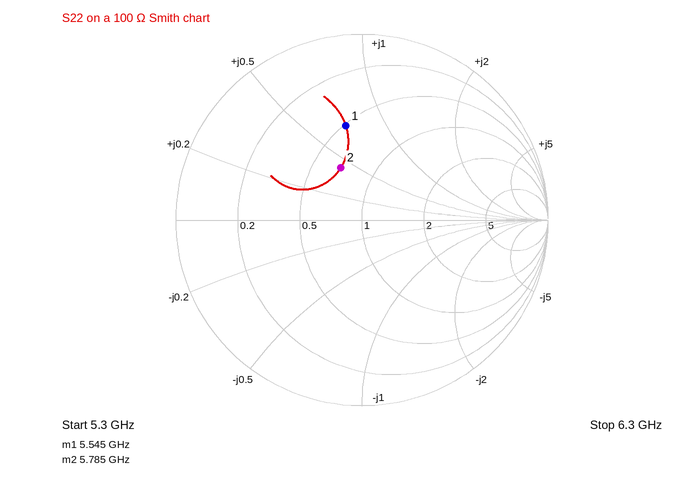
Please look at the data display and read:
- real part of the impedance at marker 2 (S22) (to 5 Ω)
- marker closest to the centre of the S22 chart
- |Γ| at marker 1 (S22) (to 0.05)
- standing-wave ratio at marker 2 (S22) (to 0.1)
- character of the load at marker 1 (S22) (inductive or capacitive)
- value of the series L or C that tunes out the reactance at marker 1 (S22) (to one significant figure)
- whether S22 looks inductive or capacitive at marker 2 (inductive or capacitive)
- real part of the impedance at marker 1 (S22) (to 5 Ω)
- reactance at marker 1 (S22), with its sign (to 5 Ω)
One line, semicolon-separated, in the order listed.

70 Ω; marker 2; 0.50; 1.9; inductive; 400 fF; inductive; 50 Ω; +70 Ω
